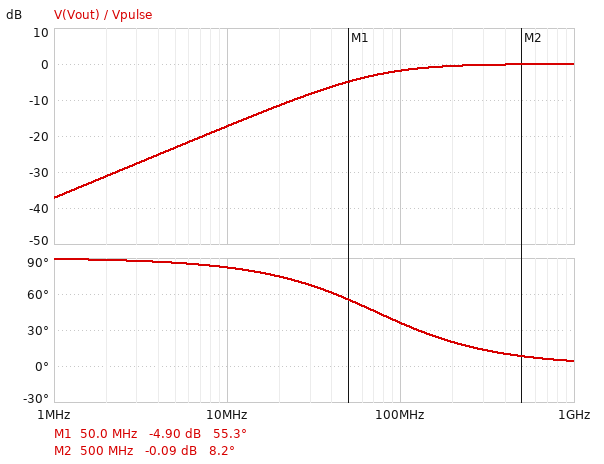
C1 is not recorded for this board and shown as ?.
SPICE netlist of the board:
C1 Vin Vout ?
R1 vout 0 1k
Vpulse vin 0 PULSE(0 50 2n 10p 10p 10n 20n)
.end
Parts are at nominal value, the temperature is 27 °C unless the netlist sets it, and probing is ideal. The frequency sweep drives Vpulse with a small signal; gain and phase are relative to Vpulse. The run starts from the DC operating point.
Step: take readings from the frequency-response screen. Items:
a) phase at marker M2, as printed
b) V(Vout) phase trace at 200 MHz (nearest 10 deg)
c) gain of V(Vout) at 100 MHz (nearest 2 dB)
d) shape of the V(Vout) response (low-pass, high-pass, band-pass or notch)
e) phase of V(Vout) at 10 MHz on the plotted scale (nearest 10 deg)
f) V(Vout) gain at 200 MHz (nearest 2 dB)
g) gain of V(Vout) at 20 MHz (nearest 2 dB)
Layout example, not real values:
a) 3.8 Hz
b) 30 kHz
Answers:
a) 8.2 deg
b) 20 deg
c) -2 dB
d) high-pass
e) 80 deg
f) 0 dB
g) -12 dB
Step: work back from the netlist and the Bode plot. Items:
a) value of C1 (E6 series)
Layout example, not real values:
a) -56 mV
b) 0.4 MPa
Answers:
a) 2.2 pF
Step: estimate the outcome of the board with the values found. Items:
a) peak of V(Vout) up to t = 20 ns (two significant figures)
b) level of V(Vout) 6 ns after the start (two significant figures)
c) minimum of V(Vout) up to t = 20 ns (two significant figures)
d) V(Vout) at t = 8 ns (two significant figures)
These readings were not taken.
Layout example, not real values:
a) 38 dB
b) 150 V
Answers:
a) 50 V
b) 8.1 V
c) -49 V
d) 3.3 V
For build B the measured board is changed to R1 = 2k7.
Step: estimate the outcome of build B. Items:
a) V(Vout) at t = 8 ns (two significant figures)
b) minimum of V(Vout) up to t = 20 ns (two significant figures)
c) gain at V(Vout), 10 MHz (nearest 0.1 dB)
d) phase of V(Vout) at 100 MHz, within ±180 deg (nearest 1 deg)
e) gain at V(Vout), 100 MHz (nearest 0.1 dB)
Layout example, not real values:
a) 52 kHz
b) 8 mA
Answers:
a) 18 V
b) -41 V
c) -9.1 dB
d) 15 deg
e) -0.3 dB
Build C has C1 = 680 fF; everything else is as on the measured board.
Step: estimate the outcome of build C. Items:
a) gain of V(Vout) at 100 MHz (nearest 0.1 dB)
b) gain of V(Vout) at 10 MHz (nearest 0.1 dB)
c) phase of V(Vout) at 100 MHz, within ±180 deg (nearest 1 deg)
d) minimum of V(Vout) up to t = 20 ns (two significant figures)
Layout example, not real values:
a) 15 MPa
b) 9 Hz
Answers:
a) -8.1 dB
b) -27.4 dB
c) 67 deg
d) -50 V
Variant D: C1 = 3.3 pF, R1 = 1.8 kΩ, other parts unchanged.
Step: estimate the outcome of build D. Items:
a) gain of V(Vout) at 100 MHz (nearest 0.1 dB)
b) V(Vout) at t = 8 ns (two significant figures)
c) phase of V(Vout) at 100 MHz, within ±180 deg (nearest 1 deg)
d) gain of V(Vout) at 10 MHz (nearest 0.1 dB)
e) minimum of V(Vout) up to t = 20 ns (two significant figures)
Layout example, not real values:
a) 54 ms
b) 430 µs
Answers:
a) -0.3 dB
b) 18 V
c) 15 deg
d) -9.1 dB
e) -41 V
